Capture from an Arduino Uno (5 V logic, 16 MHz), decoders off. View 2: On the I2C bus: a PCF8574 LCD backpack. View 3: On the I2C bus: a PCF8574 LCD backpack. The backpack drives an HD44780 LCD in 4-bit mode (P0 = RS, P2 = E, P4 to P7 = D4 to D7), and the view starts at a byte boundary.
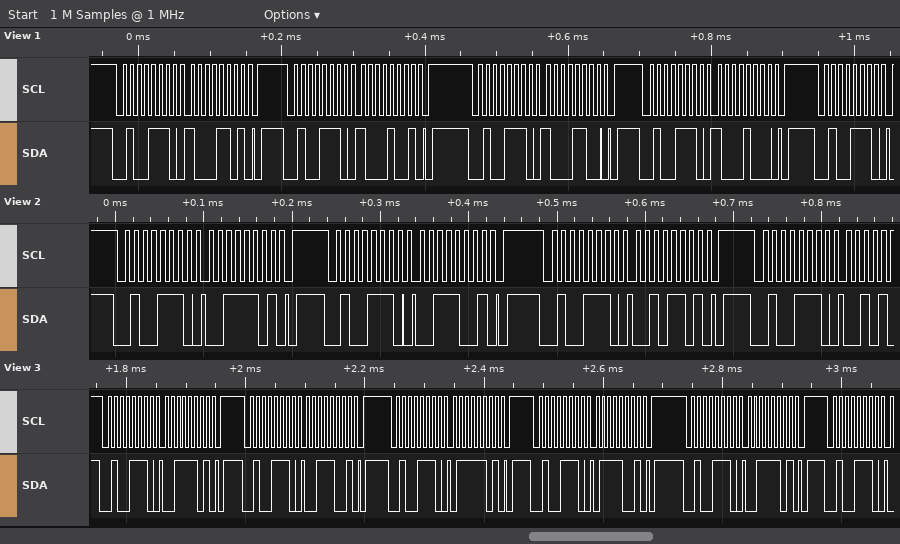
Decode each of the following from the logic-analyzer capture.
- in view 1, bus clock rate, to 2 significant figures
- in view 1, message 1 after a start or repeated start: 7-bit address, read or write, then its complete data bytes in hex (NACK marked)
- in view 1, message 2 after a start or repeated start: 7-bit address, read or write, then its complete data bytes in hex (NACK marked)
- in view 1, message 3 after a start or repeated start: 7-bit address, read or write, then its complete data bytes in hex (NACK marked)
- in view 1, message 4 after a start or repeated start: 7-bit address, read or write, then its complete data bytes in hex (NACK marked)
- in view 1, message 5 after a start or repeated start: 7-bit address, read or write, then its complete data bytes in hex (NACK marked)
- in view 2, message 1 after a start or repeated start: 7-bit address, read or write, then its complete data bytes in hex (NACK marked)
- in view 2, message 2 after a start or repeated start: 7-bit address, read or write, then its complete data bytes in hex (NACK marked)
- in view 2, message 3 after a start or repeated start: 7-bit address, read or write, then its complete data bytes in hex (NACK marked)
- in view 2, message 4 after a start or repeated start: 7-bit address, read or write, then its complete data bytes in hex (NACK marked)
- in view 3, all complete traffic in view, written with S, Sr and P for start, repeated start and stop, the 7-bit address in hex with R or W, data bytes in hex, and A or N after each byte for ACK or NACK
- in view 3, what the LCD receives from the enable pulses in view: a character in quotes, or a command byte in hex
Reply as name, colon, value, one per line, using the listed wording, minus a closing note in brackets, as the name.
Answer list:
in view 1, bus clock rate, to 2 significant figures: 100 kHz
in view 1, message 1 after a start or repeated start: 7-bit address, read or write, then its complete data bytes in hex: 0x27 write: 8D
in view 1, message 2 after a start or repeated start: 7-bit address, read or write, then its complete data bytes in hex: 0x27 write: 89
in view 1, message 3 after a start or repeated start: 7-bit address, read or write, then its complete data bytes in hex: 0x27 write: 8C
in view 1, message 4 after a start or repeated start: 7-bit address, read or write, then its complete data bytes in hex: 0x27 write: 88
in view 1, message 5 after a start or repeated start: 7-bit address, read or write, then its complete data bytes in hex: 0x27 write
in view 2, message 1 after a start or repeated start: 7-bit address, read or write, then its complete data bytes in hex: 0x27 write: 3D
in view 2, message 2 after a start or repeated start: 7-bit address, read or write, then its complete data bytes in hex: 0x27 write: 39
in view 2, message 3 after a start or repeated start: 7-bit address, read or write, then its complete data bytes in hex: 0x27 write: 2D
in view 2, message 4 after a start or repeated start: 7-bit address, read or write, then its complete data bytes in hex: 0x27 write
in view 3, all complete traffic in view, written with S, Sr and P for start, repeated start and stop, the 7-bit address in hex with R or W, data bytes in hex, and A or N after each byte for ACK or NACK: S 27W A 3D A P S 27W A 39 A P S 27W A 7D A P S 27W A 79 A P S 27W A 3D A P S 27W A
in view 3, what the LCD receives from the enable pulses in view: a character in quotes, or a command byte in hex: '7'
